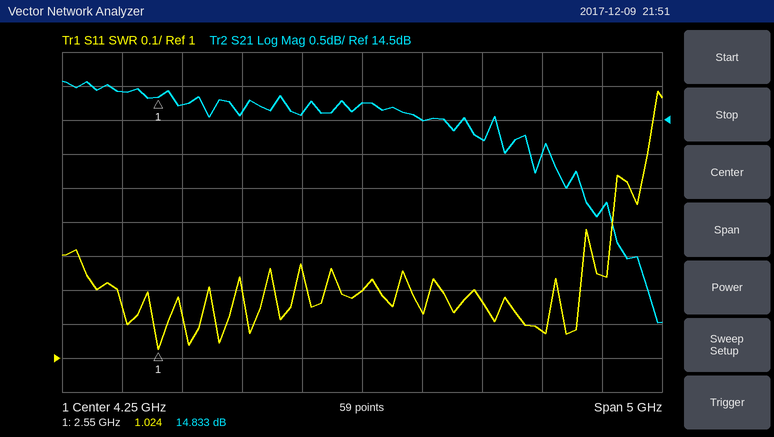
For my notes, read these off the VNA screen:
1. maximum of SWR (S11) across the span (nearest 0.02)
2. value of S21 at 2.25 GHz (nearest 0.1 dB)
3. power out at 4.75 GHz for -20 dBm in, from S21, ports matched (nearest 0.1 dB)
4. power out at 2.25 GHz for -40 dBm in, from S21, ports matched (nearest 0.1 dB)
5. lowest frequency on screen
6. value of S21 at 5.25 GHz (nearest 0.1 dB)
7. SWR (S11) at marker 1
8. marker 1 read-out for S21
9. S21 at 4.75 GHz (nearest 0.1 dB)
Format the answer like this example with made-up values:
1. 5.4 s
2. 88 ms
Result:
1. 1.78
2. 14.9 dB
3. -5.5 dBm
4. -25.1 dBm
5. 1.75 GHz
6. 14.2 dB
7. 1.024
8. 14.833 dB
9. 14.5 dB
